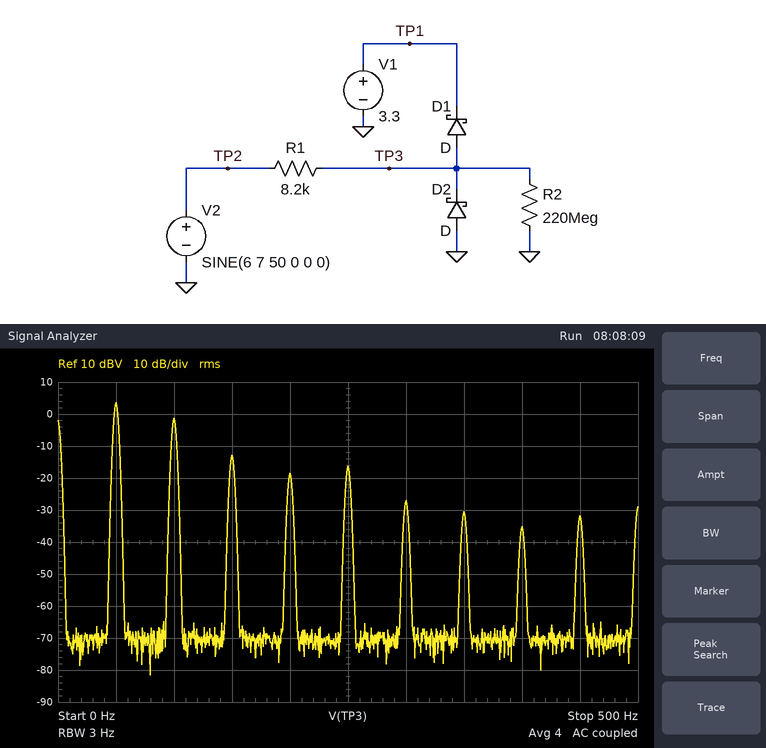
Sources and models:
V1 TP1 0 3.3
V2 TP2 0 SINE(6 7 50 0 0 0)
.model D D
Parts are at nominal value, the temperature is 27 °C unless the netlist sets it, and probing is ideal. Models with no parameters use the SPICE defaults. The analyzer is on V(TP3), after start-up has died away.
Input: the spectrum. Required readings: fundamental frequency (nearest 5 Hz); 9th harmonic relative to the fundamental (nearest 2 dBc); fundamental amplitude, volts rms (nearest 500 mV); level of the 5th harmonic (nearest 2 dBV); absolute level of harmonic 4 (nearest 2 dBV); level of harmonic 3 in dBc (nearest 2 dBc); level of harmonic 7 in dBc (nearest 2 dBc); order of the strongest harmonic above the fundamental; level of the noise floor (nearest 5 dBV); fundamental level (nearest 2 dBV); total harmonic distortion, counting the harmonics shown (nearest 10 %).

50 Hz
-36 dBc
1.5 V
-16 dBV
-18 dBV
-16 dBc
-34 dBc
2
-70 dBV
4 dBV
60 %
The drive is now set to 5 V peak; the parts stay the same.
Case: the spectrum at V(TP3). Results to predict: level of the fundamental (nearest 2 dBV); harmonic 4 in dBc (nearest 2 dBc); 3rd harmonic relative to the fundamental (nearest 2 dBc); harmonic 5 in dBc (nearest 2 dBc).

-2 dBV
-42 dBc
-12 dBc
-22 dBc
